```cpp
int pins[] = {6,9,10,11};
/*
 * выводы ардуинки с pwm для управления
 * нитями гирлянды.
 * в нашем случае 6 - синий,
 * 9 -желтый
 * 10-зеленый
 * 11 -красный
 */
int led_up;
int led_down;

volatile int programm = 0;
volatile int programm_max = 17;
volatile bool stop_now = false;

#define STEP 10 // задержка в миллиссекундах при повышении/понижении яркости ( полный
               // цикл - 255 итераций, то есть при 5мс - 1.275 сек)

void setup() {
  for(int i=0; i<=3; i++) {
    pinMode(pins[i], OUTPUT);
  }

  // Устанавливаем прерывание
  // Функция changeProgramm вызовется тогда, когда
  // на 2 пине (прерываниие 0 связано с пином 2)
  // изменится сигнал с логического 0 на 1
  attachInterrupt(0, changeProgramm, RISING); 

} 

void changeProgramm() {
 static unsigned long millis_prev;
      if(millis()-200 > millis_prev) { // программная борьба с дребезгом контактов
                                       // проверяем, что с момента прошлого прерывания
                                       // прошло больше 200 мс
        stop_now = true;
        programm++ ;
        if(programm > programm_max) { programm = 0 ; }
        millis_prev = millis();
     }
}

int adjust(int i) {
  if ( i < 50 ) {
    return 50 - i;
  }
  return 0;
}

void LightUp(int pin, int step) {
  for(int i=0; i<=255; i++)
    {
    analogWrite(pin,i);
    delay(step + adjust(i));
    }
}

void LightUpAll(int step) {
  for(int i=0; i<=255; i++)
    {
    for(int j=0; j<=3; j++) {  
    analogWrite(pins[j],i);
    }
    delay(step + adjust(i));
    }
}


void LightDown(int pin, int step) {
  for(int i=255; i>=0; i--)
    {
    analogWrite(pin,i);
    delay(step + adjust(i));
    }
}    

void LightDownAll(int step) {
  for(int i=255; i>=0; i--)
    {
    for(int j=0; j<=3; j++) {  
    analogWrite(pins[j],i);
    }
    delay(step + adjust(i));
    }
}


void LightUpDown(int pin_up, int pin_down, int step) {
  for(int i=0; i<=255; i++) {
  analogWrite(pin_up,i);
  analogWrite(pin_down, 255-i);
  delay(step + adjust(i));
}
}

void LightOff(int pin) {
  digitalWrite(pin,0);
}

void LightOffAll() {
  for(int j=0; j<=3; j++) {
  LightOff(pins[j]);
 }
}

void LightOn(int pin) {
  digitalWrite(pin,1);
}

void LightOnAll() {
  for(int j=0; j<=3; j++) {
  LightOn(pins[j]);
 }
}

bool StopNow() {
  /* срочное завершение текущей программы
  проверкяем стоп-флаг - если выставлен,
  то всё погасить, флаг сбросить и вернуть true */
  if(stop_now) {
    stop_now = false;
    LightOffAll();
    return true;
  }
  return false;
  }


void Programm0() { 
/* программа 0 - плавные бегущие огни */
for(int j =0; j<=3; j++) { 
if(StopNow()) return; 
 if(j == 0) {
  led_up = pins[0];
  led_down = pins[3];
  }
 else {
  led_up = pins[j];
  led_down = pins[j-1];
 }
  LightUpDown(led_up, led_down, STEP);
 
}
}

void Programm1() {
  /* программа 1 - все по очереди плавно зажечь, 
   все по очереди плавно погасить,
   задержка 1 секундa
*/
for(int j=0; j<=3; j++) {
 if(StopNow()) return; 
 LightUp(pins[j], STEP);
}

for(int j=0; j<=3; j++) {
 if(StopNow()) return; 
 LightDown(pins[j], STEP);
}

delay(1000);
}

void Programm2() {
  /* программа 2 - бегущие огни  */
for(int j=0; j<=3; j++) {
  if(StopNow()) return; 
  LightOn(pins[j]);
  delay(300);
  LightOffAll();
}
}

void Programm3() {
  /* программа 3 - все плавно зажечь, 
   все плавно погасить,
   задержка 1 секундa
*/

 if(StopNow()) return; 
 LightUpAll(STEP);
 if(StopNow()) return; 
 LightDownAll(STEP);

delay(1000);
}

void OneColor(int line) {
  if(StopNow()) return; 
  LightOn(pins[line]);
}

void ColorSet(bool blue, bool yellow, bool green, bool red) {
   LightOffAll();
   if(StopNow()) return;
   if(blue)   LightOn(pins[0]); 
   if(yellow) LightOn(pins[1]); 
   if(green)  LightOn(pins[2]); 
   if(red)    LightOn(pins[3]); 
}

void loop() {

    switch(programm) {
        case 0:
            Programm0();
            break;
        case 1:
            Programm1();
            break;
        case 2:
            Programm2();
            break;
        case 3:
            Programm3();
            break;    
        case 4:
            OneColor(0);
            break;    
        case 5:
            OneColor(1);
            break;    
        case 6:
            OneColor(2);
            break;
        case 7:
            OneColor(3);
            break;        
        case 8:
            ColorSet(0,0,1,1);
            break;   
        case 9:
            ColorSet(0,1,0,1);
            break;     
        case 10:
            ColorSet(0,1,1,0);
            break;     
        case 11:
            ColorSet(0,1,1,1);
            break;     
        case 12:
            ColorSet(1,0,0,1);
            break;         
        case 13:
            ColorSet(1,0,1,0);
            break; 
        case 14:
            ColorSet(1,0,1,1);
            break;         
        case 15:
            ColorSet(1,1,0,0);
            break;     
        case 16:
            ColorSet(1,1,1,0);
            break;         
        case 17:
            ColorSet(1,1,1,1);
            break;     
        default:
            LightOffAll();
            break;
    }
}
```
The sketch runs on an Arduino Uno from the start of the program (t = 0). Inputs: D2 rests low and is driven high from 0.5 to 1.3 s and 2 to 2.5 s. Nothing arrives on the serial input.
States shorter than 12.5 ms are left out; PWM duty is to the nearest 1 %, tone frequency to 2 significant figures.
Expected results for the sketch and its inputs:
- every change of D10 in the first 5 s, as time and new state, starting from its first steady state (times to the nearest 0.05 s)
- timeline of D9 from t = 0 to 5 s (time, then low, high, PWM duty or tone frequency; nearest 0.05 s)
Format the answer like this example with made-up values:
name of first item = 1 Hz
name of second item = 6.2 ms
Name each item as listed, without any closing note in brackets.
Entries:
every change of D10 in the first 5 s, as time and new state, starting from its first steady state = 0 s low; 4.45 s high; 4.75 s low
timeline of D9 from t = 0 to 5 s = 0 s low; 4.15 s high; 4.45 s low
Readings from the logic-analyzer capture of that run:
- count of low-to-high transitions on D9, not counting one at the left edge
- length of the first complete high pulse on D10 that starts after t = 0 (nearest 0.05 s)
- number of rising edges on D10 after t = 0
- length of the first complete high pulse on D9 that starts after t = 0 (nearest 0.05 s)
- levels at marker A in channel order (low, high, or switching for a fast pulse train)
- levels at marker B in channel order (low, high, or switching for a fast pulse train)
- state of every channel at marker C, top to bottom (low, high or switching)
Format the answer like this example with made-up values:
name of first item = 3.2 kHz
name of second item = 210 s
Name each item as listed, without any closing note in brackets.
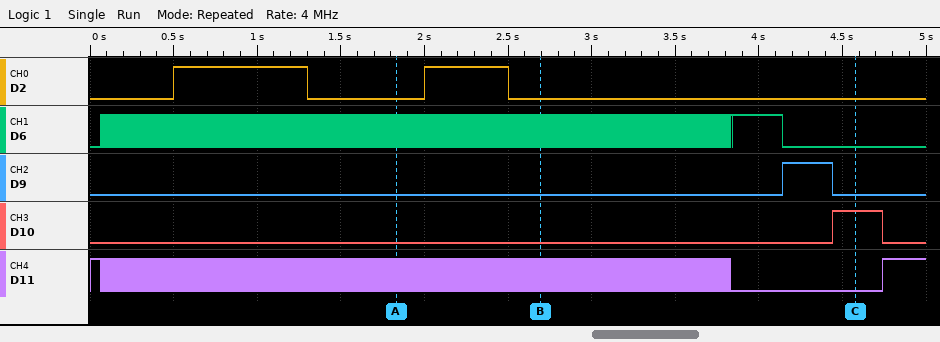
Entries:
count of low-to-high transitions on D9, not counting one at the left edge = 1
length of the first complete high pulse on D10 that starts after t = 0 = 0.30 s
number of rising edges on D10 after t = 0 = 1
length of the first complete high pulse on D9 that starts after t = 0 = 0.30 s
levels at marker A in channel order = D2 low, D6 switching, D9 low, D10 low, D11 switching
levels at marker B in channel order = D2 low, D6 switching, D9 low, D10 low, D11 switching
state of every channel at marker C, top to bottom = D2 low, D6 low, D9 low, D10 high, D11 low
